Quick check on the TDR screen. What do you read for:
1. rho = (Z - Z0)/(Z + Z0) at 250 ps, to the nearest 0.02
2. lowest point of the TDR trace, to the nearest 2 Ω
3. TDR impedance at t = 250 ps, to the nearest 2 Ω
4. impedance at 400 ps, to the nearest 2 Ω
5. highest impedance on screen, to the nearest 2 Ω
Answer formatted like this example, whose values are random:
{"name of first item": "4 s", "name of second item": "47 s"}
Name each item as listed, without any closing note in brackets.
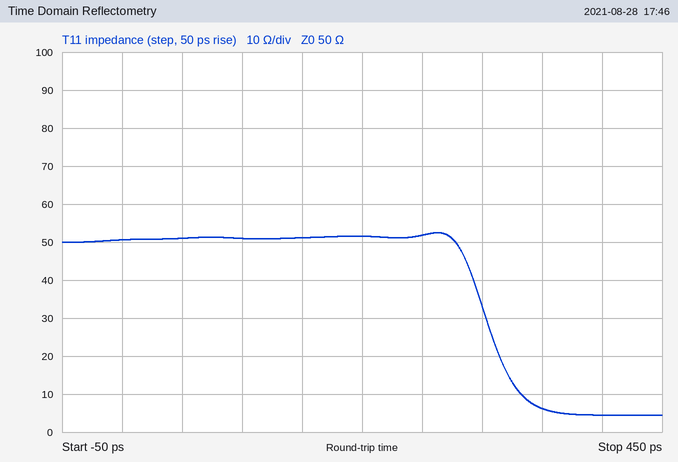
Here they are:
{"rho = (Z - Z0)/(Z + Z0) at 250 ps, to the nearest 0.02": "+0.02", "lowest point of the TDR trace, to the nearest 2 Ω": "4 Ω", "TDR impedance at t = 250 ps, to the nearest 2 Ω": "52 Ω", "impedance at 400 ps, to the nearest 2 Ω": "4 Ω", "highest impedance on screen, to the nearest 2 Ω": "52 Ω"}
